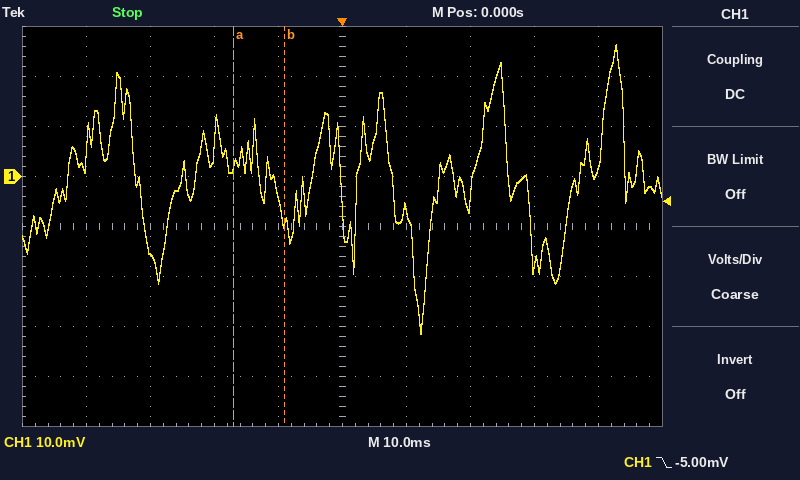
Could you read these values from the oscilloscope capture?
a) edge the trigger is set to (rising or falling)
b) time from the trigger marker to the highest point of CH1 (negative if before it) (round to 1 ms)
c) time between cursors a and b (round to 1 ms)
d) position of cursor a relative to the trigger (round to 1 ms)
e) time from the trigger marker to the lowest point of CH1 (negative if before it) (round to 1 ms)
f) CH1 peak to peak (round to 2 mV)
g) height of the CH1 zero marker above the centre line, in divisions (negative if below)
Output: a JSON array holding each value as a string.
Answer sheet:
["falling", "+43 ms", "8 ms", "-17 ms", "+12 ms", "58 mV", "+1.0 div"]
